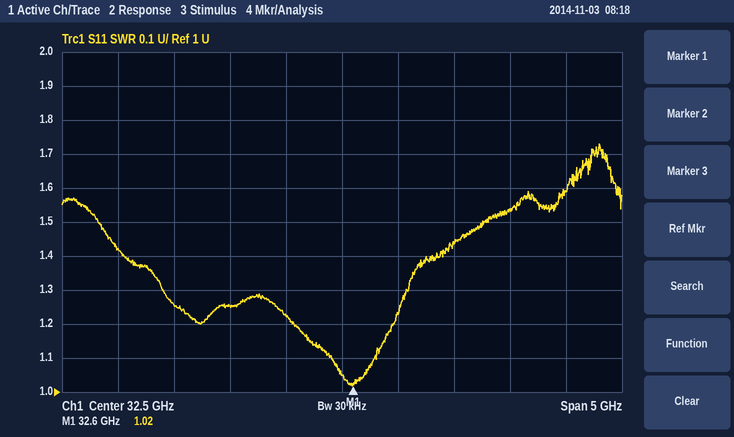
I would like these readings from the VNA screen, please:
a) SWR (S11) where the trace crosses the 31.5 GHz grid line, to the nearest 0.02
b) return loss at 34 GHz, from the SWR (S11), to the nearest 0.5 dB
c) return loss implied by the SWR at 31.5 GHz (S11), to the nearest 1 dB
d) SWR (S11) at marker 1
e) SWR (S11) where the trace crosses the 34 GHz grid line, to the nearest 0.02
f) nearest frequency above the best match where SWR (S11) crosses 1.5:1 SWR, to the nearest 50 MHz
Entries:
1.26
13.5 dB
19 dB
1.02
1.54
33.75 GHz
